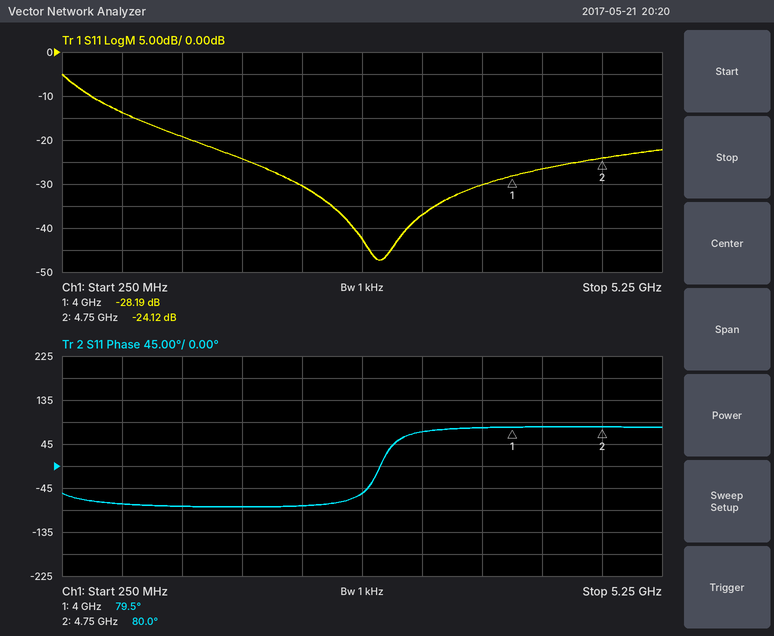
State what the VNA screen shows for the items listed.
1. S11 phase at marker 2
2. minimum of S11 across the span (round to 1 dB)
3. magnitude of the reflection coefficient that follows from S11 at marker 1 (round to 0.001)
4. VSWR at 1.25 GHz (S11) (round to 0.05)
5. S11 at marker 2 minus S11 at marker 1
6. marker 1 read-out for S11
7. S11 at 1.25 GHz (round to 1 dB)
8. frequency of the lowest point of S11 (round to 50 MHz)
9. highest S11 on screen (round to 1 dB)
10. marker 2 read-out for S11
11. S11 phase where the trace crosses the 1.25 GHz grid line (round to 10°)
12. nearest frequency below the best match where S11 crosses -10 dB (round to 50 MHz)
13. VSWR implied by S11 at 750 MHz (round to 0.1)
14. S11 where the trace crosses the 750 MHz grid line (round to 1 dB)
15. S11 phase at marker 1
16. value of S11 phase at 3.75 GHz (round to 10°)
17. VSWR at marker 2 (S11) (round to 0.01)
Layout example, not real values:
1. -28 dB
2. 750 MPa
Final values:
1. 80.0°
2. -47 dB
3. 0.039
4. 1.25
5. 4.07 dB
6. -28.19 dB
7. -19 dB
8. 2.90 GHz
9. -5 dB
10. -24.12 dB
11. -80°
12. 500 MHz
13. 1.5
14. -14 dB
15. 79.5°
16. 80°
17. 1.13
